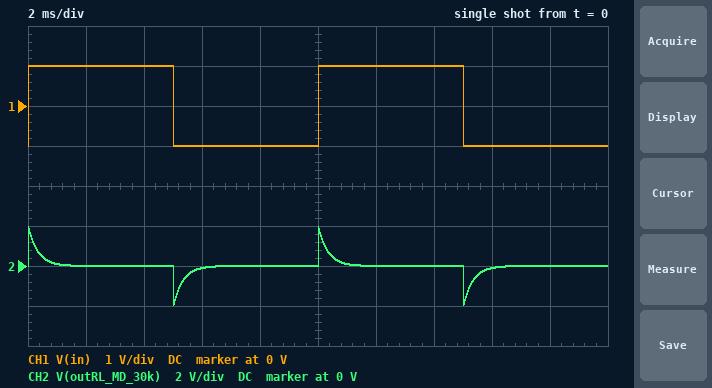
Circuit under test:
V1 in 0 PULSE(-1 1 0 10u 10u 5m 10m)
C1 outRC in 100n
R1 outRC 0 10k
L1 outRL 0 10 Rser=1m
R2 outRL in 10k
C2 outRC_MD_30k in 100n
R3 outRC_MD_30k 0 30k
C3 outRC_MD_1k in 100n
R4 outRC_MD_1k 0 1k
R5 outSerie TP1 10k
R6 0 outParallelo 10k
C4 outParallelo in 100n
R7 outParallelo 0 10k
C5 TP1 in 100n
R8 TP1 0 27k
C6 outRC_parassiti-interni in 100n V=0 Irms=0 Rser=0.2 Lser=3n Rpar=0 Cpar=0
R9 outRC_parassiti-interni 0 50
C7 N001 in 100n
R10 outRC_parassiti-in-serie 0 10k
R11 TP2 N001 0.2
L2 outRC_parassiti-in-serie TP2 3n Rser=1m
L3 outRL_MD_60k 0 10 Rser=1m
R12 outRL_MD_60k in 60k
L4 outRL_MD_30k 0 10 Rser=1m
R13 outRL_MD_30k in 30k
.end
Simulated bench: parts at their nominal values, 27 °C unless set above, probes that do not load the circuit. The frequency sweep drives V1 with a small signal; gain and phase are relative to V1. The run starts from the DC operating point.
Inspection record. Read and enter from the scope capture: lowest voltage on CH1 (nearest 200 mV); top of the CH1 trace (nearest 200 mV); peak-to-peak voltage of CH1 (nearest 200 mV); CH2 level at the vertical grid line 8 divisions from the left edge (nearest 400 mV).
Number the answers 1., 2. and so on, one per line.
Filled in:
1. -1.0 V
2. 1.0 V
3. 2.0 V
4. 0 V
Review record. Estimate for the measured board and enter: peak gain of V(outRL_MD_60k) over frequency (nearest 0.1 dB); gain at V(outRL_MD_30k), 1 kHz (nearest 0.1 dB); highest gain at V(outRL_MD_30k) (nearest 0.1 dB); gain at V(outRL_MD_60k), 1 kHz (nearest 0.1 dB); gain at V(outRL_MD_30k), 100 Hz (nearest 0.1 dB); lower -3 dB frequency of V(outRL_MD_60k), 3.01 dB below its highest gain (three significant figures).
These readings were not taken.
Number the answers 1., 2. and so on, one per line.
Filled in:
1. 0 dB
2. -0.9 dB
3. 0 dB
4. -2.8 dB
5. -13.8 dB
6. 955 Hz
